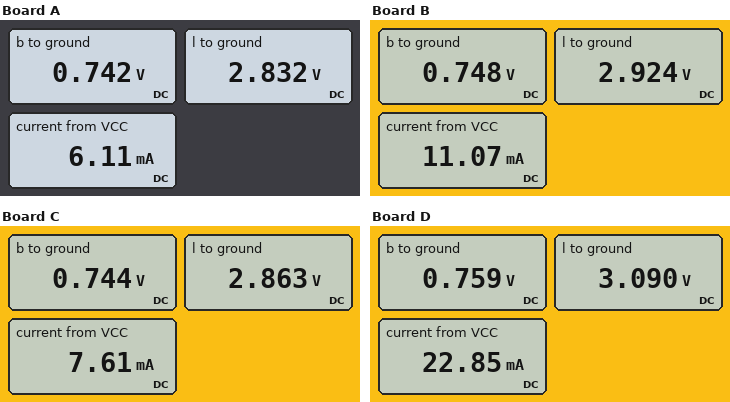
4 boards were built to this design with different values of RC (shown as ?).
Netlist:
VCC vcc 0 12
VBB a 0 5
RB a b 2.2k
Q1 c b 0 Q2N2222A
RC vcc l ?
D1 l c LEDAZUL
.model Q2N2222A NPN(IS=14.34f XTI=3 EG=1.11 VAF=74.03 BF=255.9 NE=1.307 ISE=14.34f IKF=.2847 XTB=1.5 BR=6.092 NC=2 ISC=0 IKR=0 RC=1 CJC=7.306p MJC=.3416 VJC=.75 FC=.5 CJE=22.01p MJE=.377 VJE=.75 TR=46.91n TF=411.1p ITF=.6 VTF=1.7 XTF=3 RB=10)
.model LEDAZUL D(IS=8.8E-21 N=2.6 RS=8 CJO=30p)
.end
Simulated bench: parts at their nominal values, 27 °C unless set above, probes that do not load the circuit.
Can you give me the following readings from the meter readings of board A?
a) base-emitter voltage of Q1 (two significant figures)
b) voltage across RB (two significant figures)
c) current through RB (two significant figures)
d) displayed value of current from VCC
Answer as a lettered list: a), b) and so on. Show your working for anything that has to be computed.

a) 742 mV = 740 mV
b) 5 V - 742 mV = 4.3 V
c) (5 V - 742 mV) / 2.2 kΩ = 1.9 mA
d) 6.11 mA
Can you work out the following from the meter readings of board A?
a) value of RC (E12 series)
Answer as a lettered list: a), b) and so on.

a) 1.5 kΩ
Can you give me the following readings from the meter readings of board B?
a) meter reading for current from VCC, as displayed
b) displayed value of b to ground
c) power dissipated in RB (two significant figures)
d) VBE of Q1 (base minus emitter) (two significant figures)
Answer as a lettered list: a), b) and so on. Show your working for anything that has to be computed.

a) 11.07 mA
b) 0.748 V
c) (5 V - 748 mV)^2 / 2.2 kΩ = 8.2 mW
d) 748 mV = 750 mV
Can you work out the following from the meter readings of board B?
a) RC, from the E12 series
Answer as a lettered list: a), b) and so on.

a) 820 Ω
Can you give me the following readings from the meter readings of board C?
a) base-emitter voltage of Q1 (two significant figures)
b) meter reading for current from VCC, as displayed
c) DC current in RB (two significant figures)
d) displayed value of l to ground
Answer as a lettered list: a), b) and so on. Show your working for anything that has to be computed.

a) 744 mV = 740 mV
b) 7.61 mA
c) (5 V - 744 mV) / 2.2 kΩ = 1.9 mA
d) 2.863 V
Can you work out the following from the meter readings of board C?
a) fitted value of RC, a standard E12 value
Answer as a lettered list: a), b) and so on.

a) 1.2 kΩ
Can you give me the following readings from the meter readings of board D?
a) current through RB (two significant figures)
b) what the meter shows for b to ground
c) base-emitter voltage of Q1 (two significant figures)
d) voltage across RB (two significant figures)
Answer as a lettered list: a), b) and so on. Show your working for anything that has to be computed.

a) (5 V - 759 mV) / 2.2 kΩ = 1.9 mA
b) 0.759 V
c) 759 mV = 760 mV
d) 5 V - 759 mV = 4.2 V
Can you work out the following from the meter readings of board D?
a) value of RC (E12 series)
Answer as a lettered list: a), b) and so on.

a) 390 Ω
